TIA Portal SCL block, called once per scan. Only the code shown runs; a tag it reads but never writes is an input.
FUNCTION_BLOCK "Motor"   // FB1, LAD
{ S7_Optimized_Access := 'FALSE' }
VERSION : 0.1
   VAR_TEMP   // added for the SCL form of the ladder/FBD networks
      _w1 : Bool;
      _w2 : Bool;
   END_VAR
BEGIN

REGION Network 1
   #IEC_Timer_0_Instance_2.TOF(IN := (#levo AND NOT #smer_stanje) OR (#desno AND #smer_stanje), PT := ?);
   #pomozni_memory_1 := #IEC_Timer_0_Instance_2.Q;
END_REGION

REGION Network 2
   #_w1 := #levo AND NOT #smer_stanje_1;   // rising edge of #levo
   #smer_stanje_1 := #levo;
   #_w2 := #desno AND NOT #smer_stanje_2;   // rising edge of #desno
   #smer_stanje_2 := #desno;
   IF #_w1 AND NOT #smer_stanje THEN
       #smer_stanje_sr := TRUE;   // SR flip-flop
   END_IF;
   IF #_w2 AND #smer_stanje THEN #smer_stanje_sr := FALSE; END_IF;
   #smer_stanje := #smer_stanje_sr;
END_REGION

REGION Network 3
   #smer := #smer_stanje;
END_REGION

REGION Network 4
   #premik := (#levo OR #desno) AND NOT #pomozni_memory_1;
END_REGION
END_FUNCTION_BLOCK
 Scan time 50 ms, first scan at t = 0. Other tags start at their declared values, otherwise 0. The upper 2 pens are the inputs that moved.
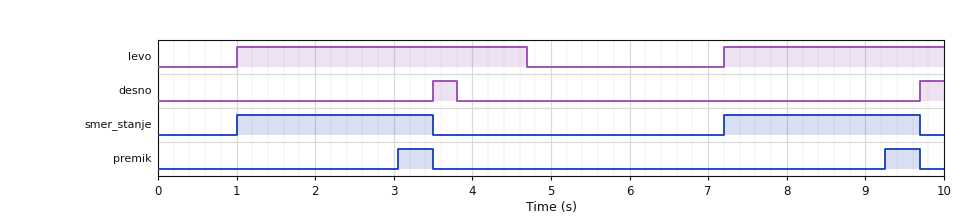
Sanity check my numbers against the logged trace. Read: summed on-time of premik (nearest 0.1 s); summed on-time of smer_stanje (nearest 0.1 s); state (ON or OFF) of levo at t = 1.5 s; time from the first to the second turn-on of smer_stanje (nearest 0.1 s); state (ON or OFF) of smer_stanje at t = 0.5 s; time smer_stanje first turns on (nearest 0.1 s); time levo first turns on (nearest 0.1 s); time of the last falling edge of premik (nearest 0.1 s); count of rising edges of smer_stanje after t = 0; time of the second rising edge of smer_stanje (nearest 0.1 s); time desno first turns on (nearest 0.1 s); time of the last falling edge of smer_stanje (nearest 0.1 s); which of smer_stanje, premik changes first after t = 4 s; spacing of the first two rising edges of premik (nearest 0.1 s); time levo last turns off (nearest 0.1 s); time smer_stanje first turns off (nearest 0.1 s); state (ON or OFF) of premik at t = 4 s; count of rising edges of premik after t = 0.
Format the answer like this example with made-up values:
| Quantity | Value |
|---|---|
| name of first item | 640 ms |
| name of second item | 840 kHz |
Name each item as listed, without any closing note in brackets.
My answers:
| Quantity | Value |
|---|---|
| summed on-time of premik | 0.9 s |
| summed on-time of smer_stanje | 5.0 s |
| state (ON or OFF) of levo at t = 1.5 s | ON |
| time from the first to the second turn-on of smer_stanje | 6.2 s |
| state (ON or OFF) of smer_stanje at t = 0.5 s | OFF |
| time smer_stanje first turns on | 1.0 s |
| time levo first turns on | 1.0 s |
| time of the last falling edge of premik | 9.7 s |
| count of rising edges of smer_stanje after t = 0 | 2 |
| time of the second rising edge of smer_stanje | 7.2 s |
| time desno first turns on | 3.5 s |
| time of the last falling edge of smer_stanje | 9.7 s |
| which of smer_stanje, premik changes first after t = 4 s | smer_stanje |
| spacing of the first two rising edges of premik | 6.2 s |
| time levo last turns off | 4.7 s |
| time smer_stanje first turns off | 3.5 s |
| state (ON or OFF) of premik at t = 4 s | OFF |
| count of rising edges of premik after t = 0 | 2 |
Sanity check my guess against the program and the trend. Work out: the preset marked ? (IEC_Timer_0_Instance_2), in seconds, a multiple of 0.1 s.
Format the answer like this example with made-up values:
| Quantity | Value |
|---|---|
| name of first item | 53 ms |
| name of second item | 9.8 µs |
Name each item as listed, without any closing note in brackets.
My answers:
| Quantity | Value |
|---|---|
| the preset marked ? (IEC_Timer_0_Instance_2), in seconds, a multiple of 0.1 s | 2.0 s |
